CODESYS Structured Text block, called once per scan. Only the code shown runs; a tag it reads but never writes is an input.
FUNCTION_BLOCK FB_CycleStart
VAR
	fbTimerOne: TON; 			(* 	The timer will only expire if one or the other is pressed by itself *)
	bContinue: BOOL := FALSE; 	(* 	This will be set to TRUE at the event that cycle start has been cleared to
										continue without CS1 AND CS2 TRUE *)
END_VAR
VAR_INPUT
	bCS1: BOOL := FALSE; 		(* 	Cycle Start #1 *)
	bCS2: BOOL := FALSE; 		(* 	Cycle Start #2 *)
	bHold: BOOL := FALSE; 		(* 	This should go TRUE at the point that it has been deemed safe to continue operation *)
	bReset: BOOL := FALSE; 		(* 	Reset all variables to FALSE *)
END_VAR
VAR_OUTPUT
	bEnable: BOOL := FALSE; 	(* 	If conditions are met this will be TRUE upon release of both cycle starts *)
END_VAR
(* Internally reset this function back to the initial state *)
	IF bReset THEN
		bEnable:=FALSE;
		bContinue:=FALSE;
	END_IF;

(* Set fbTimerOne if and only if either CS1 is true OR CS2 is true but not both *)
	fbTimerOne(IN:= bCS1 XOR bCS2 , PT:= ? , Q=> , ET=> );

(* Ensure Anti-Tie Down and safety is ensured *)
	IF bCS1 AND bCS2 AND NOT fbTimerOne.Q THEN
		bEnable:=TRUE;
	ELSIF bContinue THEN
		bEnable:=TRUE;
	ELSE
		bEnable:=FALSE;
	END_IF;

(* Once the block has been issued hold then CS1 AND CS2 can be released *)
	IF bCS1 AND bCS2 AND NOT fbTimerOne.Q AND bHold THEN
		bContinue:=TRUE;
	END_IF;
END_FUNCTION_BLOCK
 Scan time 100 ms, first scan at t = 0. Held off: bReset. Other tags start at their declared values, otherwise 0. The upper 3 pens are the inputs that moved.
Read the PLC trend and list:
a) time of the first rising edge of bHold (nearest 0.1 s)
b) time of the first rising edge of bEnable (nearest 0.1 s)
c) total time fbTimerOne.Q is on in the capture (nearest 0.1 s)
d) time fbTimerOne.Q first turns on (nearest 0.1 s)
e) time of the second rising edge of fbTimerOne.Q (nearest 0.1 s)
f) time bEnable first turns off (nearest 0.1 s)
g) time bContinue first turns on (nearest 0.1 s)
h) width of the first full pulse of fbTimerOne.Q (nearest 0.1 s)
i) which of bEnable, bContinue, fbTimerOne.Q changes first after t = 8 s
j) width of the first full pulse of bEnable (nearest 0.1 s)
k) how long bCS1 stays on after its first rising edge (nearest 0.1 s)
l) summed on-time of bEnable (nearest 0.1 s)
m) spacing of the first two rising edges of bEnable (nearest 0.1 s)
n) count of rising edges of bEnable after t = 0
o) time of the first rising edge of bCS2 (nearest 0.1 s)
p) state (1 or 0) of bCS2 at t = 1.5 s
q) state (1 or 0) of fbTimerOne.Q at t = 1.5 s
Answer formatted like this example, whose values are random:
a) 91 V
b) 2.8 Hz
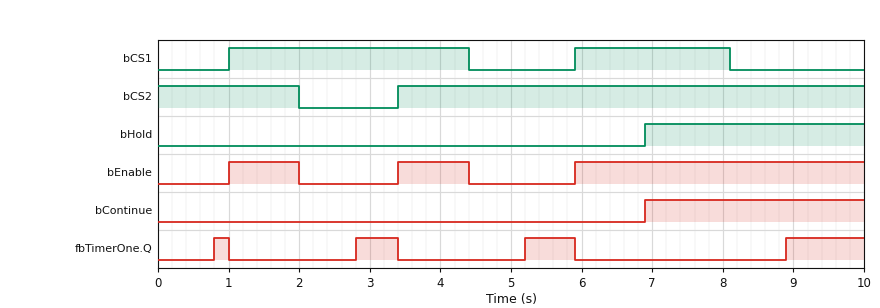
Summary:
a) 6.9 s
b) 1.0 s
c) 2.6 s
d) 0.8 s
e) 2.8 s
f) 2.0 s
g) 6.9 s
h) 0.2 s
i) fbTimerOne.Q
j) 1.0 s
k) 3.4 s
l) 6.1 s
m) 2.4 s
n) 3
o) 3.4 s
p) 1
q) 0
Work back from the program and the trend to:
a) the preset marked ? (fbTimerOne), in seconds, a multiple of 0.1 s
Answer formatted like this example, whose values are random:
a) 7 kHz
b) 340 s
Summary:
a) 0.8 s
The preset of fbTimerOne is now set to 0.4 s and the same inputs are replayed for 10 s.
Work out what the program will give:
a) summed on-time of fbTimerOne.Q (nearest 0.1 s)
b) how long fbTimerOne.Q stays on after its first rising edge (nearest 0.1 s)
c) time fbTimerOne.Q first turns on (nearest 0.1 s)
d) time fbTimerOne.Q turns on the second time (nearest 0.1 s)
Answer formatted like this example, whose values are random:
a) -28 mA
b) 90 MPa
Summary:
a) 4.2 s
b) 0.6 s
c) 0.4 s
d) 2.4 s
